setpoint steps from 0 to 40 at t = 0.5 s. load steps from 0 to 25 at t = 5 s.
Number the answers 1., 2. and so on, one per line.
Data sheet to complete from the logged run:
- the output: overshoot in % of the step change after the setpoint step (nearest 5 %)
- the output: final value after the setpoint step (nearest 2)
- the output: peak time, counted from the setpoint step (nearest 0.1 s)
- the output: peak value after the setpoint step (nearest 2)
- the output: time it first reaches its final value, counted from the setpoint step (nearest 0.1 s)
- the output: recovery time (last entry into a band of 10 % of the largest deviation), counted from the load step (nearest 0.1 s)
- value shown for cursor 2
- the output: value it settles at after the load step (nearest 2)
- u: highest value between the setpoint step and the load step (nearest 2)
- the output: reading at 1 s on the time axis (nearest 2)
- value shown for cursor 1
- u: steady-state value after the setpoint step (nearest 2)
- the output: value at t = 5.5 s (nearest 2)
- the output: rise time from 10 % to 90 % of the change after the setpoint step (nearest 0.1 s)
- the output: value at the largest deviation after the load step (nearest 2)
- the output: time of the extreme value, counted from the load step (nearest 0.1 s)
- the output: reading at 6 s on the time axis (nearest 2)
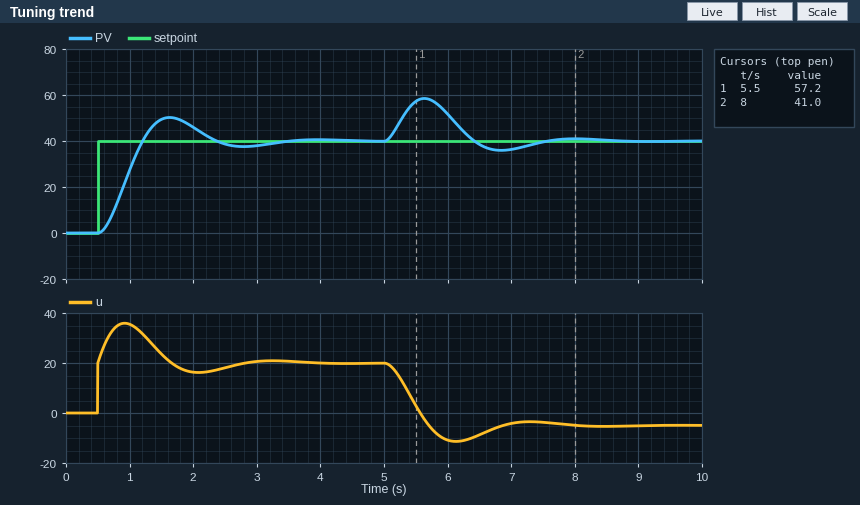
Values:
1. 25 %
2. 40
3. 1.1 s
4. 50
5. 0.7 s
6. 2.3 s
7. 41.0
8. 40
9. 36
10. 28
11. 57.2
12. 20
13. 58
14. 0.5 s
15. 58
16. 0.6 s
17. 52
